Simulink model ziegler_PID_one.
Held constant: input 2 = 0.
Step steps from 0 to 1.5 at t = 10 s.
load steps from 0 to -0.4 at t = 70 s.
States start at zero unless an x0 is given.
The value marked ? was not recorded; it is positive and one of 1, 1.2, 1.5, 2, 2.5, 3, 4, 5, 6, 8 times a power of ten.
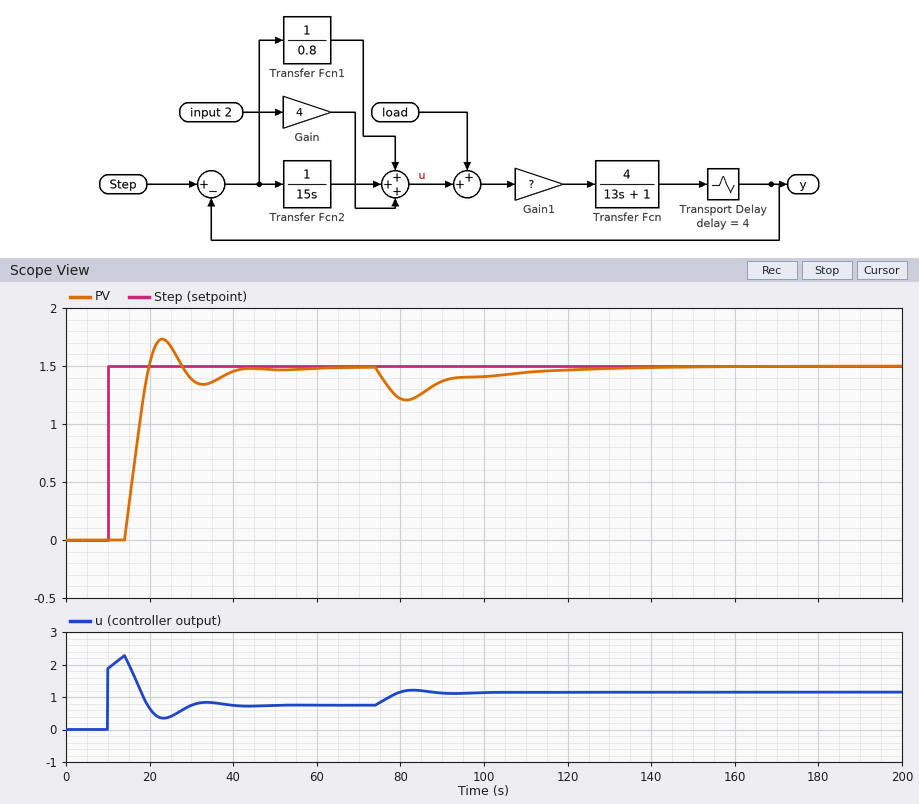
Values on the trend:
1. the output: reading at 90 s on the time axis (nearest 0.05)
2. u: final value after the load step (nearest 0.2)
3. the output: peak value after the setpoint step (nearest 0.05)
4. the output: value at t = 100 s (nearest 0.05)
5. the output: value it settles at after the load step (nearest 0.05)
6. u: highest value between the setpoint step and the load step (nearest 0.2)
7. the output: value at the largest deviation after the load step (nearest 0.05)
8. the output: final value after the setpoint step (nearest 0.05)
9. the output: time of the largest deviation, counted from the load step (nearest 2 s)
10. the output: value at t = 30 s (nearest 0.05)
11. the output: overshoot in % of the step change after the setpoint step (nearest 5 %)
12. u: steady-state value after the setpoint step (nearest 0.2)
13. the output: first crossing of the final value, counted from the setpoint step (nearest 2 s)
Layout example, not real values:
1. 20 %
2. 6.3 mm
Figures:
1. 1.35
2. 1.2
3. 1.75
4. 1.40
5. 1.50
6. 2.2
7. 1.20
8. 1.50
9. 12 s
10. 1.40
11. 15 %
12. 0.8
13. 10 s
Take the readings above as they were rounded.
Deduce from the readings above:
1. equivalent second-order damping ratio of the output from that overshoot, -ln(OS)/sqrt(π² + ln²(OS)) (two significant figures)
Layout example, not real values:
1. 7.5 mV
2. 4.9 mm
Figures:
1. 0.52
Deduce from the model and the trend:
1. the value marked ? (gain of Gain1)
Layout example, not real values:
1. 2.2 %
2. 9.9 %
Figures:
1. 0.5
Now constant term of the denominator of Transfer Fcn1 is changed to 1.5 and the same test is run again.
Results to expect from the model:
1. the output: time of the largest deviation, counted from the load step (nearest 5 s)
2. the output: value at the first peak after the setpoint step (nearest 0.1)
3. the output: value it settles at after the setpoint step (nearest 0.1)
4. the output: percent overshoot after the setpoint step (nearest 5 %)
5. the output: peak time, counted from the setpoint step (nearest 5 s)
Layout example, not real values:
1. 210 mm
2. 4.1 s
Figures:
1. 15 s
2. 1.6
3. 1.5
4. 10 %
5. 25 s
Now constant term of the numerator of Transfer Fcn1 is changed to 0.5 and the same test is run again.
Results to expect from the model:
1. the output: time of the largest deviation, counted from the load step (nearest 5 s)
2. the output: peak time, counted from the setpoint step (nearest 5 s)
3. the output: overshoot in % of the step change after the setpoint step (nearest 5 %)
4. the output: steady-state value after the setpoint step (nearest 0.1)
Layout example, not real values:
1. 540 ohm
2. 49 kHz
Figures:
1. 15 s
2. 25 s
3. 10 %
4. 1.5
